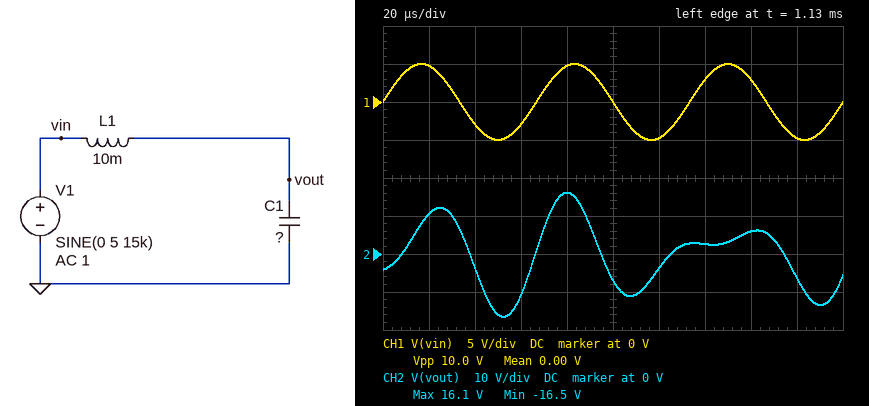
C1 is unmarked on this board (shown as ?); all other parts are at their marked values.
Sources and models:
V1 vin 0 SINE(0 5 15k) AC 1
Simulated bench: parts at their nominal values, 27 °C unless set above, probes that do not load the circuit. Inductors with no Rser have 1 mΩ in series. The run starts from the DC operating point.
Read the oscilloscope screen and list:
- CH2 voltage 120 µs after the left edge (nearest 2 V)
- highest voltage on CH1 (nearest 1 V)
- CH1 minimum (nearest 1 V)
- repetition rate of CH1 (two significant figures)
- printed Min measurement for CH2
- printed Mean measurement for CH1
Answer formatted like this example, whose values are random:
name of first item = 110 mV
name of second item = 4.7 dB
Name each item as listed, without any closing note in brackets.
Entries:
CH2 voltage 120 µs after the left edge = -4 V
highest voltage on CH1 = 5 V
CH1 minimum = -5 V
repetition rate of CH1 = 15 kHz
printed Min measurement for CH2 = -16.5 V
printed Mean measurement for CH1 = 0.00 V
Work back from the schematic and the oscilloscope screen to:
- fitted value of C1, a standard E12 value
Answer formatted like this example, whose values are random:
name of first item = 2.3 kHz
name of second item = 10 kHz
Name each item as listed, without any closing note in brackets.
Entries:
fitted value of C1, a standard E12 value = 5.6 nF
